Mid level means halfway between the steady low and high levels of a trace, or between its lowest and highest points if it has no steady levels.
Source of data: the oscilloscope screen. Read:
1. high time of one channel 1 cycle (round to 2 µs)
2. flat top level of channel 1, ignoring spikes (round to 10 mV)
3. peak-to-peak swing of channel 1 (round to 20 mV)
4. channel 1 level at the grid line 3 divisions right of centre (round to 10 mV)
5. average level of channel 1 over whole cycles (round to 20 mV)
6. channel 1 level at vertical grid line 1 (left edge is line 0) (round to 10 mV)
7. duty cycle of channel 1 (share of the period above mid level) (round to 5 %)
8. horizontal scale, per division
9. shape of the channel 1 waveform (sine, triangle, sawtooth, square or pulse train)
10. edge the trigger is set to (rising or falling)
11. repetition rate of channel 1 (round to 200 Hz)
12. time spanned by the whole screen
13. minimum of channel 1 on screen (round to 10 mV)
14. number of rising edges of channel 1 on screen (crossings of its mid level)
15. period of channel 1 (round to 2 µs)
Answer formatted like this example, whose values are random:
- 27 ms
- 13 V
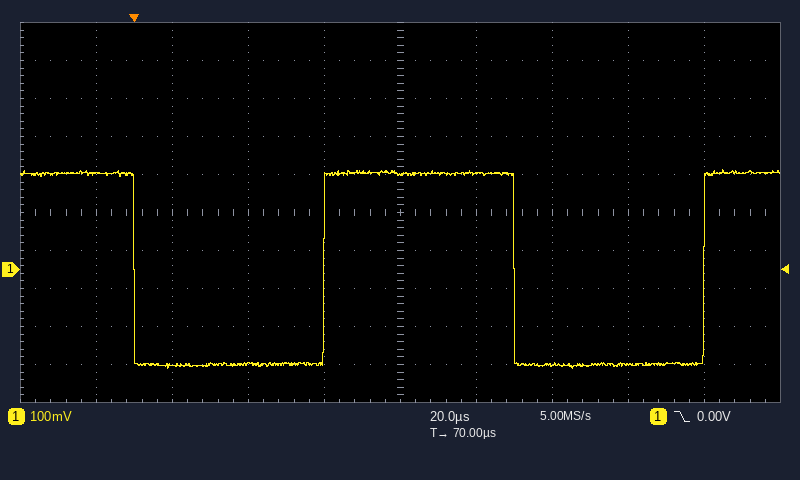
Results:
- 50 µs
- 250 mV
- 520 mV
- -250 mV
- 0 mV
- 250 mV
- 50 %
- 20 µs
- square
- falling
- 10.0 kHz
- 200 µs
- -260 mV
- 2
- 100 µs
